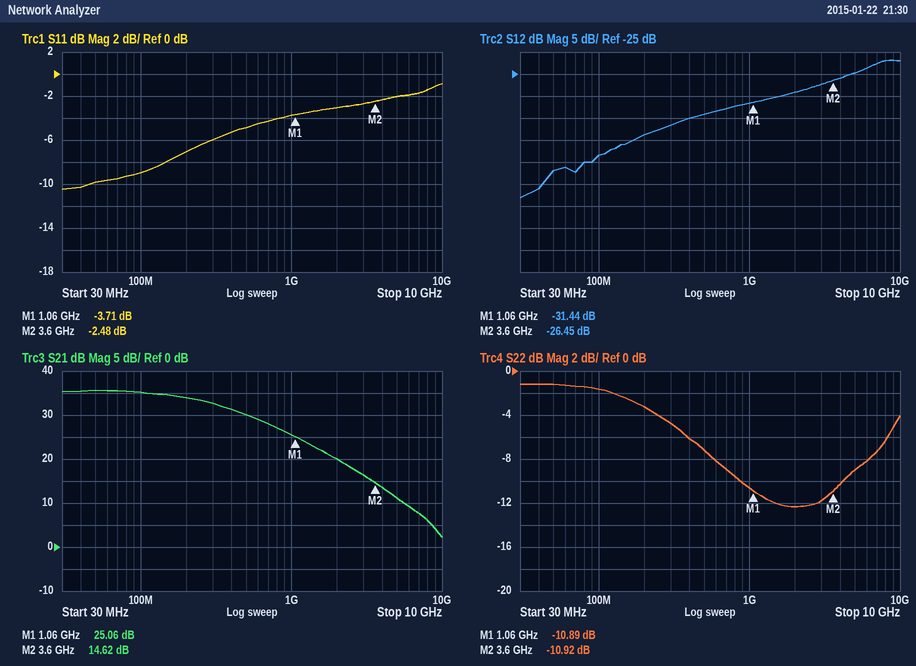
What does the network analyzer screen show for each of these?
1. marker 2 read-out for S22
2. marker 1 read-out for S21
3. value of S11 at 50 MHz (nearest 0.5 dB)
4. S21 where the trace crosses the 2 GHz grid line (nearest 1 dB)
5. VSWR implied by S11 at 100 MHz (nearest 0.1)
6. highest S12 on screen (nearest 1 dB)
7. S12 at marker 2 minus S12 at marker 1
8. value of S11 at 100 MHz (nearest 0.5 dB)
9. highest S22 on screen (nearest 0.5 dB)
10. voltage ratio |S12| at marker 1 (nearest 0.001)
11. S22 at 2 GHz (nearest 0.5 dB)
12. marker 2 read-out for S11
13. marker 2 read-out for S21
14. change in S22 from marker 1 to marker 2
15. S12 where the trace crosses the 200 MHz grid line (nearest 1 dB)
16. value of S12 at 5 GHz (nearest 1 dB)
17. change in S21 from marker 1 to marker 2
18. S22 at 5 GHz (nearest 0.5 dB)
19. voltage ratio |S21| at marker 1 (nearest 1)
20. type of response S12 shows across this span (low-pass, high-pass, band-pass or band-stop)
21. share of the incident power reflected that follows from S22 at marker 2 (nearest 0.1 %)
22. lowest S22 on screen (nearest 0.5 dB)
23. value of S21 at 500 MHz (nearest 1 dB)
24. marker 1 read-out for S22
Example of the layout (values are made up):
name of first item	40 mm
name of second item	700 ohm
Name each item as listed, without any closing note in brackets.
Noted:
marker 2 read-out for S22	-10.92 dB
marker 1 read-out for S21	25.06 dB
value of S11 at 50 MHz	-10.0 dB
S21 where the trace crosses the 2 GHz grid line	20 dB
VSWR implied by S11 at 100 MHz	2.1
highest S12 on screen	-22 dB
S12 at marker 2 minus S12 at marker 1	4.99 dB
value of S11 at 100 MHz	-9.0 dB
highest S22 on screen	-1.0 dB
voltage ratio |S12| at marker 1	0.027
S22 at 2 GHz	-12.5 dB
marker 2 read-out for S11	-2.48 dB
marker 2 read-out for S21	14.62 dB
change in S22 from marker 1 to marker 2	-0.03 dB
S12 where the trace crosses the 200 MHz grid line	-39 dB
value of S12 at 5 GHz	-25 dB
change in S21 from marker 1 to marker 2	-10.44 dB
S22 at 5 GHz	-9.0 dB
voltage ratio |S21| at marker 1	18
type of response S12 shows across this span	high-pass
share of the incident power reflected that follows from S22 at marker 2	8.1 %
lowest S22 on screen	-12.5 dB
value of S21 at 500 MHz	30 dB
marker 1 read-out for S22	-10.89 dB
